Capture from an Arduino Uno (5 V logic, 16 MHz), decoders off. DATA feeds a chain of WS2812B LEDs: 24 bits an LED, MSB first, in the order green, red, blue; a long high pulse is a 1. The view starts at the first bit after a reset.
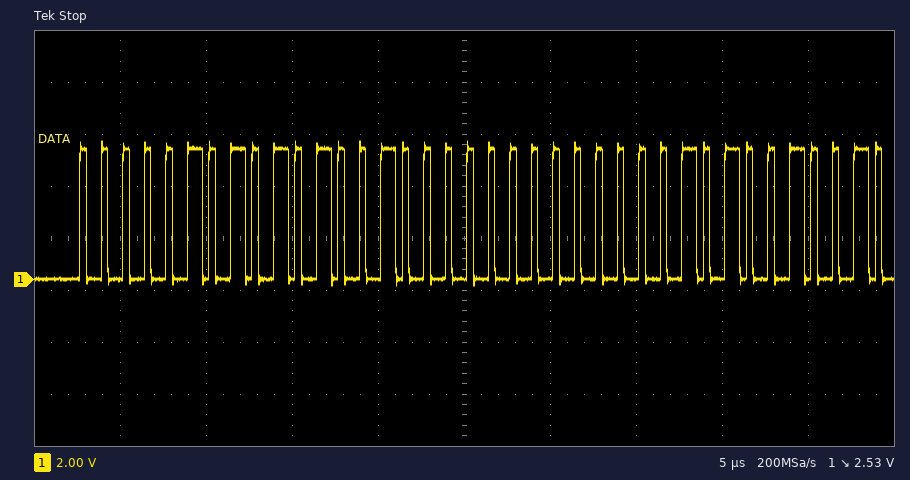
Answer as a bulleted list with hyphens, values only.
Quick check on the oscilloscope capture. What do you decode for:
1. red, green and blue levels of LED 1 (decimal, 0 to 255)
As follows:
- 82, 5, 0
